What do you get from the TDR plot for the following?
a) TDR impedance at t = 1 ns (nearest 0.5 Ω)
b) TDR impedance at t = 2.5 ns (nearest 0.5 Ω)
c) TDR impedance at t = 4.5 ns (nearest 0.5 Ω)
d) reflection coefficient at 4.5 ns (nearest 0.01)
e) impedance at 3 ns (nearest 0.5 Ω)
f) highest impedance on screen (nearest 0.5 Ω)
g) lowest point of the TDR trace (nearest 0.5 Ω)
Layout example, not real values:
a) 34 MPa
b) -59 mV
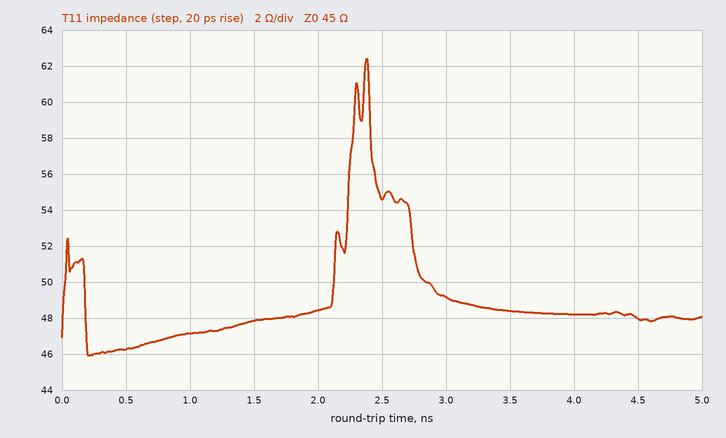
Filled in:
a) 47.0 Ω
b) 54.5 Ω
c) 48.0 Ω
d) +0.03
e) 49.0 Ω
f) 62.5 Ω
g) 46.0 Ω
